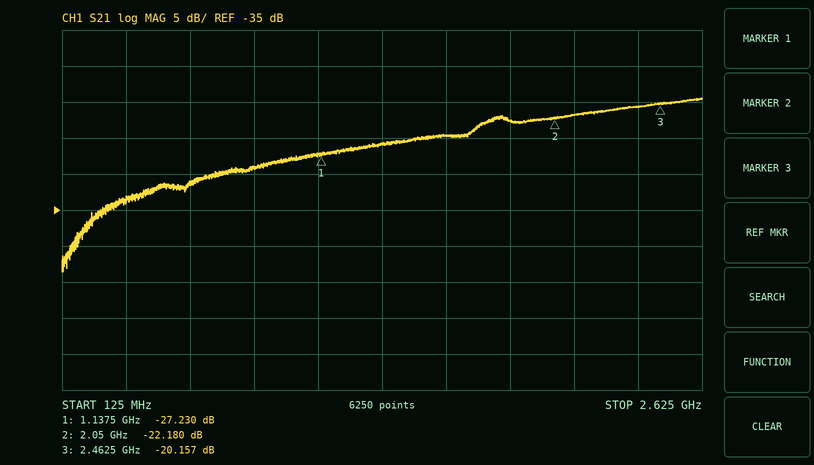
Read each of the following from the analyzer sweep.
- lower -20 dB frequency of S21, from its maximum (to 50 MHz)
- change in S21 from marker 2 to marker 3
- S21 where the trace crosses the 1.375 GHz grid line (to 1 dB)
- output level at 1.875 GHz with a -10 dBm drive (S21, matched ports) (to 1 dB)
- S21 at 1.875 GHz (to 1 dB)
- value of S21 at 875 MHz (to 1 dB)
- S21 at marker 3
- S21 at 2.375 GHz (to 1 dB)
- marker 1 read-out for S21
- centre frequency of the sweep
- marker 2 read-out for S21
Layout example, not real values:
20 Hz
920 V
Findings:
200 MHz
2.023 dB
-26 dB
-33 dBm
-23 dB
-29 dB
-20.157 dB
-21 dB
-27.230 dB
1.375 GHz
-22.180 dB
